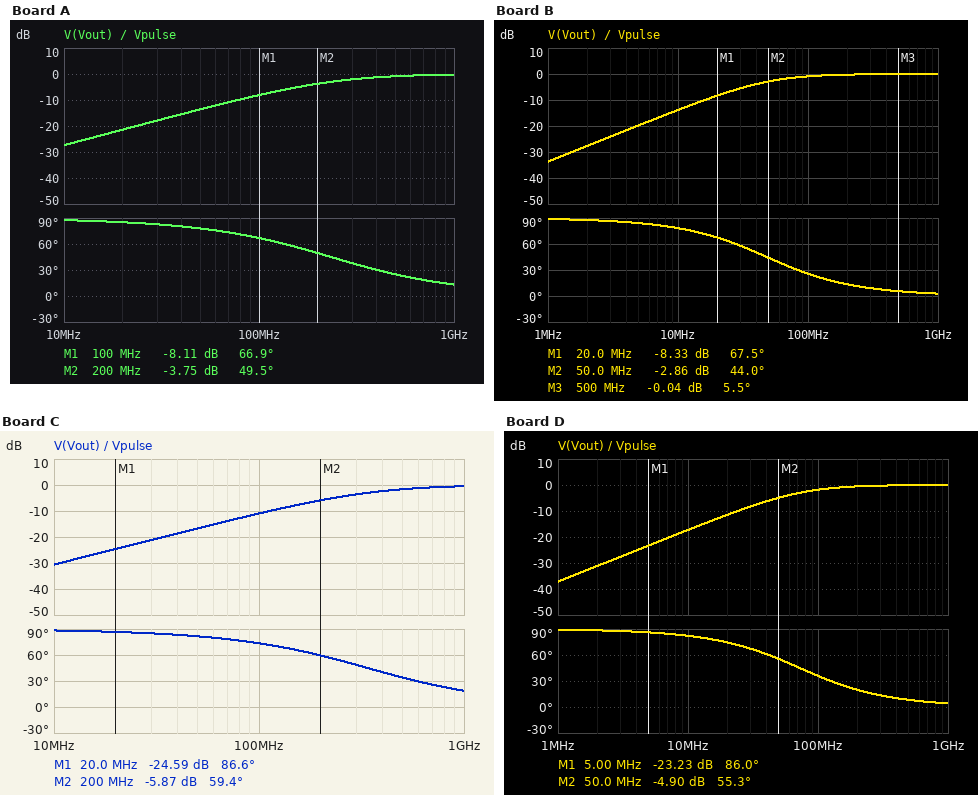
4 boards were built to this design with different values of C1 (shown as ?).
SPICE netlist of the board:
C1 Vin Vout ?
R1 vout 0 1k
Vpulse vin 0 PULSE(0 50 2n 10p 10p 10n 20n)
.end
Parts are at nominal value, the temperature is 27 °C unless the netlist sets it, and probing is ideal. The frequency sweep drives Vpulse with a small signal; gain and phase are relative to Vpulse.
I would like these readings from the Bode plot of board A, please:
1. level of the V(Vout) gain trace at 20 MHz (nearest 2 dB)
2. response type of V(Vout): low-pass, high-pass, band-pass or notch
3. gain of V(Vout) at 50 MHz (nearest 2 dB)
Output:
-22 dB
high-pass
-14 dB
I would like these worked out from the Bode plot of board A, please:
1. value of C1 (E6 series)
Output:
680 fF
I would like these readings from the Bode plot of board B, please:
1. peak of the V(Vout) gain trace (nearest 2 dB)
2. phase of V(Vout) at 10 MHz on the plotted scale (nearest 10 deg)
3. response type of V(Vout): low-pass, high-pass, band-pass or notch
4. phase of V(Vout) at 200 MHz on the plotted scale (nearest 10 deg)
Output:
0 dB
80 deg
high-pass
10 deg
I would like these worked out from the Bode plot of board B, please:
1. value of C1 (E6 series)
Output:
3.3 pF
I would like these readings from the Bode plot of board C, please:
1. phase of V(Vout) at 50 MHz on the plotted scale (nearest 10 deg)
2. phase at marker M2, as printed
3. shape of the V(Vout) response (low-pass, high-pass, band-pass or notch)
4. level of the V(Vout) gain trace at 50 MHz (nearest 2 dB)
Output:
80 deg
59.4 deg
high-pass
-16 dB
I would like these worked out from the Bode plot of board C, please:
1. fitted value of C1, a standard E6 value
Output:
470 fF
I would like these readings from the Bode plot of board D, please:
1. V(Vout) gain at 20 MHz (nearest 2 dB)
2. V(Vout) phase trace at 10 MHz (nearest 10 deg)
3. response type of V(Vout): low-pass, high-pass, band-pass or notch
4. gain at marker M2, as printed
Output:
-12 dB
80 deg
high-pass
-4.90 dB
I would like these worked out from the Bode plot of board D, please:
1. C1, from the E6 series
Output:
2.2 pF
